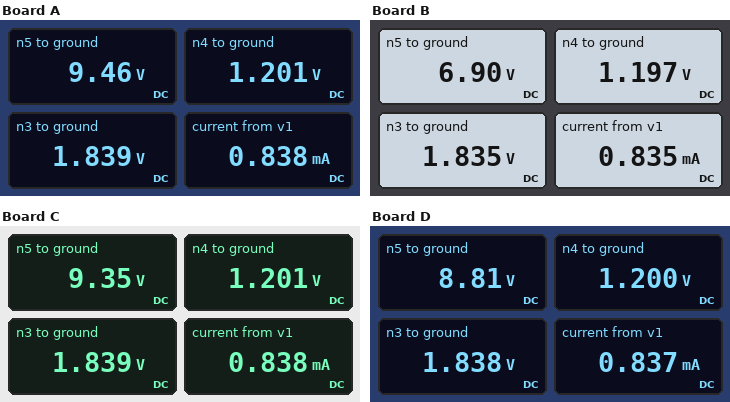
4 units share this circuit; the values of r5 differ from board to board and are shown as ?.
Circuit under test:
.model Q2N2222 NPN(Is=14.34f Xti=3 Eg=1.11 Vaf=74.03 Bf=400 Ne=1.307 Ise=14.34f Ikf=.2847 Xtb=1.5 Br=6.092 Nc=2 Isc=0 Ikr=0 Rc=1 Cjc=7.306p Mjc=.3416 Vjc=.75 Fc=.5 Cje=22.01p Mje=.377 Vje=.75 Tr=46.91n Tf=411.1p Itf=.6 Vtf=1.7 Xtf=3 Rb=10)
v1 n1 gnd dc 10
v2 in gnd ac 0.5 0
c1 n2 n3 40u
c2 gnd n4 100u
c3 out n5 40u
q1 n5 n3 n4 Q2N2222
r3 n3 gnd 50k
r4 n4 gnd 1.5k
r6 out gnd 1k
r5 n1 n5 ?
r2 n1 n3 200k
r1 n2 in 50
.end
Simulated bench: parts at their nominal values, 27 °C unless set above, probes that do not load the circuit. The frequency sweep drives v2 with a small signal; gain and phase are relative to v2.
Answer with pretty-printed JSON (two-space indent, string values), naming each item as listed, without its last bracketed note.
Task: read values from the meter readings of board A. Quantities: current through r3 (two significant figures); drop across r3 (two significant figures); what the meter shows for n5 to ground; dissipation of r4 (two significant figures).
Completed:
{
  "current through r3": "37 µA",
  "drop across r3": "1.8 V",
  "what the meter shows for n5 to ground": "9.46 V",
  "dissipation of r4": "960 µW"
}
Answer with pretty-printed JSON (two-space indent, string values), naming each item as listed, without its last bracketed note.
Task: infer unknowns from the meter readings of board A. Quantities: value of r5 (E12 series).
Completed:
{
  "value of r5": "680 Ω"
}
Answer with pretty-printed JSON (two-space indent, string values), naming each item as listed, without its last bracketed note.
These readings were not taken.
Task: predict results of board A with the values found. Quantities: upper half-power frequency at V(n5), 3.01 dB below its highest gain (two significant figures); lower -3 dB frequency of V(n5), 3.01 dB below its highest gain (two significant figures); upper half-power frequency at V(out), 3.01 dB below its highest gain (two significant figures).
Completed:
{
  "upper half-power frequency at V(n5), 3.01 dB below its highest gain": "26 MHz",
  "lower -3 dB frequency of V(n5), 3.01 dB below its highest gain": "50 Hz",
  "upper half-power frequency at V(out), 3.01 dB below its highest gain": "26 MHz"
}
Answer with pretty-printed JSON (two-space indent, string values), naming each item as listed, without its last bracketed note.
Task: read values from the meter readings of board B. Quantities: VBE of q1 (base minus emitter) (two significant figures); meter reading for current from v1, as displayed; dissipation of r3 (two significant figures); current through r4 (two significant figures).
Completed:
{
  "VBE of q1 (base minus emitter)": "640 mV",
  "meter reading for current from v1, as displayed": "0.835 mA",
  "dissipation of r3": "67 µW",
  "current through r4": "800 µA"
}
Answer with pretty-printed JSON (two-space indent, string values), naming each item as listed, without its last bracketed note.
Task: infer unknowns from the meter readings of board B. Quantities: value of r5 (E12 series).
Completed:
{
  "value of r5": "3.9 kΩ"
}
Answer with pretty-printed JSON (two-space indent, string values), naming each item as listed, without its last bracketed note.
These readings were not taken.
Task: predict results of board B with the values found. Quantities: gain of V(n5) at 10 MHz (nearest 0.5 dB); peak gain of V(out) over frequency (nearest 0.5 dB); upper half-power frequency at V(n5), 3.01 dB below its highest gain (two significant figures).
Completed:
{
  "gain of V(n5) at 10 MHz": "26.0 dB",
  "peak gain of V(out) over frequency": "27.5 dB",
  "upper half-power frequency at V(n5), 3.01 dB below its highest gain": "15 MHz"
}
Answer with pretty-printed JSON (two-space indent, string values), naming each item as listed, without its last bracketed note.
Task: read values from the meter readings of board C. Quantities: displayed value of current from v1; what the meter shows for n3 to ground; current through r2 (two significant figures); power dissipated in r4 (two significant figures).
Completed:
{
  "displayed value of current from v1": "0.838 mA",
  "what the meter shows for n3 to ground": "1.839 V",
  "current through r2": "41 µA",
  "power dissipated in r4": "960 µW"
}
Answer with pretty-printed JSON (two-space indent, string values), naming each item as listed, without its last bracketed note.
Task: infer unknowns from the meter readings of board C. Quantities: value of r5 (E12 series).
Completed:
{
  "value of r5": "820 Ω"
}
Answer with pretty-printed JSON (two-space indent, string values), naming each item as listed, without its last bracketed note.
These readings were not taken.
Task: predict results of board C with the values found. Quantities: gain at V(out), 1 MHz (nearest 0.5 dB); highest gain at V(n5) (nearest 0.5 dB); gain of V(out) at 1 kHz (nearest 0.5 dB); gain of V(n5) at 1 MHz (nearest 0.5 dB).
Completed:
{
  "gain at V(out), 1 MHz": "22.5 dB",
  "highest gain at V(n5)": "22.5 dB",
  "gain of V(out) at 1 kHz": "22.5 dB",
  "gain of V(n5) at 1 MHz": "22.5 dB"
}
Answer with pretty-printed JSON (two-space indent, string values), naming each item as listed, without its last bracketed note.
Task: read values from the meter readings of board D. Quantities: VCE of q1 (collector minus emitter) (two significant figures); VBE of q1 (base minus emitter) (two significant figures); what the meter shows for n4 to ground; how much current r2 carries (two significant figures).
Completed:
{
  "VCE of q1 (collector minus emitter)": "7.6 V",
  "VBE of q1 (base minus emitter)": "640 mV",
  "what the meter shows for n4 to ground": "1.200 V",
  "how much current r2 carries": "41 µA"
}
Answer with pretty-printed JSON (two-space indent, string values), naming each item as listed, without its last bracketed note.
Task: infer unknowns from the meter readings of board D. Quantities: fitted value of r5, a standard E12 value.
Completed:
{
  "fitted value of r5, a standard E12 value": "1.5 kΩ"
}
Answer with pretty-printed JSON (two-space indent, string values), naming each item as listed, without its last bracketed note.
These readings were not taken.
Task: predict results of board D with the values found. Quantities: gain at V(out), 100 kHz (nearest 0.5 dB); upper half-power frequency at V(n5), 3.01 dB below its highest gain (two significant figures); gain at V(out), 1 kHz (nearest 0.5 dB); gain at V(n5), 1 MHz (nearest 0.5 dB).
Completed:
{
  "gain at V(out), 100 kHz": "25.0 dB",
  "upper half-power frequency at V(n5), 3.01 dB below its highest gain": "20 MHz",
  "gain at V(out), 1 kHz": "25.0 dB",
  "gain at V(n5), 1 MHz": "25.0 dB"
}
